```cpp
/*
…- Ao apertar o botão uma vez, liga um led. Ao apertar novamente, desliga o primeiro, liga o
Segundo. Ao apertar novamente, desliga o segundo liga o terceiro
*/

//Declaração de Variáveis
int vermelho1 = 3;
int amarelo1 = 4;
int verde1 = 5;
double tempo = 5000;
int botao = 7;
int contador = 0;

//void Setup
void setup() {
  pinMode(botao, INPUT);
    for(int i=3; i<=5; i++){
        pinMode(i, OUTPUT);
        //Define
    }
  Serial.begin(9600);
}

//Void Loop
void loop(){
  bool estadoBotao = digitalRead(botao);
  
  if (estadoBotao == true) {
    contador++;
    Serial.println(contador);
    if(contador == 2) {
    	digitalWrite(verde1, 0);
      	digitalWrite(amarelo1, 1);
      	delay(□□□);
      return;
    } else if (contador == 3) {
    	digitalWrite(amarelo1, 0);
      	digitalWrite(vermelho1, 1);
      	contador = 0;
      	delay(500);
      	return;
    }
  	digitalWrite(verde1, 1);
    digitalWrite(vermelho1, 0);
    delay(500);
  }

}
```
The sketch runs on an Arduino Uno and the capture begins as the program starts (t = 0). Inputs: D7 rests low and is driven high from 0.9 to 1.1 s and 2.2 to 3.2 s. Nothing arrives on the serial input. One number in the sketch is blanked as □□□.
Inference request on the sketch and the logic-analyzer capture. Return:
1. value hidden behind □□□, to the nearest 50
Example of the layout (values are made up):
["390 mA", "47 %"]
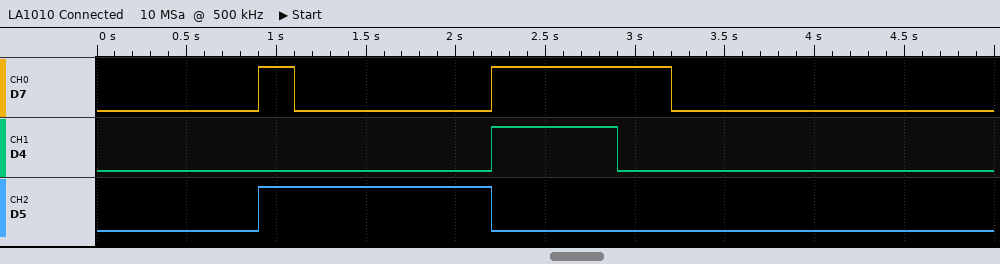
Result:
["700"]
